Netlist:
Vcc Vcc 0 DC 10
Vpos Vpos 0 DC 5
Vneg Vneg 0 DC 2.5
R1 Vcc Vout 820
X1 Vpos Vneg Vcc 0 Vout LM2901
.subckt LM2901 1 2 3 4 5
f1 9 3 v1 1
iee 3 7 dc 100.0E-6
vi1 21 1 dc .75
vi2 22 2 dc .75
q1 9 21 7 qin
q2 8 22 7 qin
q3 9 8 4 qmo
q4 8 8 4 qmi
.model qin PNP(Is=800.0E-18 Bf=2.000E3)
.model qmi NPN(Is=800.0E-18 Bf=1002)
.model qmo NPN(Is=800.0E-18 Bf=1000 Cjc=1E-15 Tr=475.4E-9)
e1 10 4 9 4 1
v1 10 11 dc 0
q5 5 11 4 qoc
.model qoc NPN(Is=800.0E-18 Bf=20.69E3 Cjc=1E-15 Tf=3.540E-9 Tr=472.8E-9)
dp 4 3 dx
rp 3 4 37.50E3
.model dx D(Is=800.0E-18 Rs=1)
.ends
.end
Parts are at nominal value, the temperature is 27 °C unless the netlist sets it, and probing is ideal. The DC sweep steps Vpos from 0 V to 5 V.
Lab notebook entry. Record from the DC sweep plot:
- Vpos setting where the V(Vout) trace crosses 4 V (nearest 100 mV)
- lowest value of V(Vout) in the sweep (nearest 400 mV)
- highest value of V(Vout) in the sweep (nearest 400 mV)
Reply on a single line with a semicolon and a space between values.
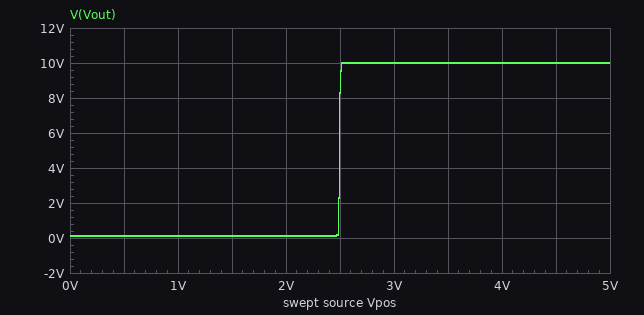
2.5 V; 0 V; 10.0 V
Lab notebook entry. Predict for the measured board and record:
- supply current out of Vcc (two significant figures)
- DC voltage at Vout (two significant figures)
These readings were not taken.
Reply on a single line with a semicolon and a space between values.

370 µA; 10 V
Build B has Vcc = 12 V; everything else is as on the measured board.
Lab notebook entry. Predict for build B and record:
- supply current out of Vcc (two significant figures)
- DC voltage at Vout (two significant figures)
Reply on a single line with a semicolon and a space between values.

420 µA; 12 V
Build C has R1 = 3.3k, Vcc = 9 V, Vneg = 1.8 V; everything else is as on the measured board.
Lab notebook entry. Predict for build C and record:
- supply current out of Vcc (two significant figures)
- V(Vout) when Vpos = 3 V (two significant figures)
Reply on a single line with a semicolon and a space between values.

340 µA; 9.0 V
